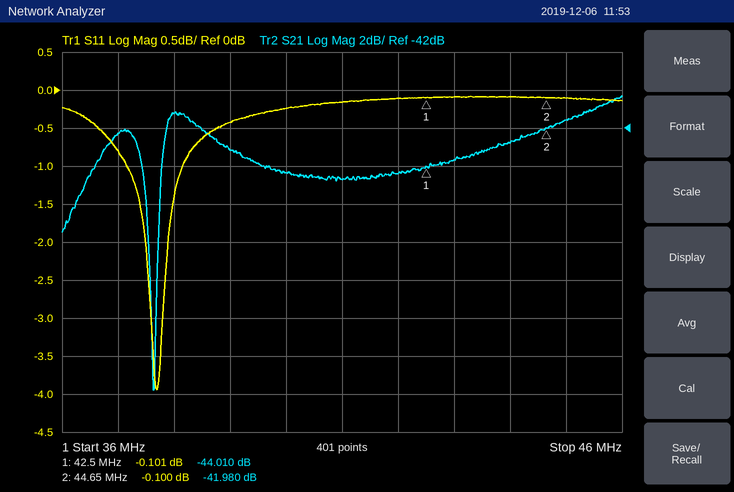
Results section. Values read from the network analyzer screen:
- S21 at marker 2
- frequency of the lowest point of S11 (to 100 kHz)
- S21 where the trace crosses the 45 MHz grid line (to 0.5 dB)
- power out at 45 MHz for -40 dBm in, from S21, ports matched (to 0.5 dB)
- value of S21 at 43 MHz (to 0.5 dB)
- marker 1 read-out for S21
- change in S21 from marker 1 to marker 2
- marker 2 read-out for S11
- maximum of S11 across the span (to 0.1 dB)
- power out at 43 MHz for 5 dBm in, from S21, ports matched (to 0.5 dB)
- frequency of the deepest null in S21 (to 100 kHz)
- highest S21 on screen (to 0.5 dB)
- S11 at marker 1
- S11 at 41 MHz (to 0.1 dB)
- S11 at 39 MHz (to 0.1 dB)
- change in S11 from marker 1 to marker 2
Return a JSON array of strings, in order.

["-41.980 dB", "37.7 MHz", "-41.5 dB", "-81.5 dBm", "-43.5 dB", "-44.010 dB", "2.030 dB", "-0.100 dB", "-0.1 dB", "-38.5 dBm", "37.6 MHz", "-40.5 dB", "-0.101 dB", "-0.2 dB", "-0.4 dB", "0.001 dB"]
